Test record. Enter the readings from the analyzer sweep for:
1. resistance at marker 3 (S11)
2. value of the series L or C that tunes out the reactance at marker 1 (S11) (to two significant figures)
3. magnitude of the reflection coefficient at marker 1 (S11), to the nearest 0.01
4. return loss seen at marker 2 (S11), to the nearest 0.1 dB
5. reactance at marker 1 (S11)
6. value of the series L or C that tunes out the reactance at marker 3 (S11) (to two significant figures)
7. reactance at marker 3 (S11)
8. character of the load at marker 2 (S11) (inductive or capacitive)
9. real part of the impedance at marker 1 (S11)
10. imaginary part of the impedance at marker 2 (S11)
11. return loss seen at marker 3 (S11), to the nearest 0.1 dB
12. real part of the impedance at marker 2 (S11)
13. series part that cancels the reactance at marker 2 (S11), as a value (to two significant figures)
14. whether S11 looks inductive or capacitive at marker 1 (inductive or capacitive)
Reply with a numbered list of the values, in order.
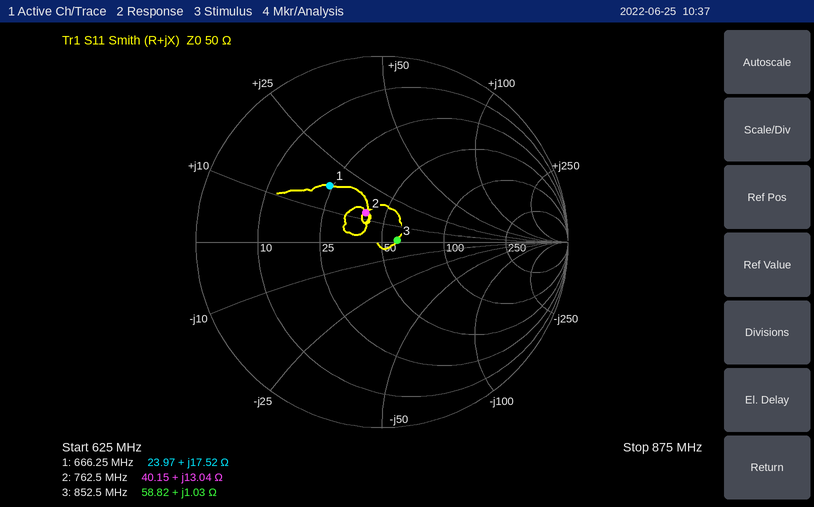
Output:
1. 58.82 Ω
2. 14 pF
3. 0.41
4. 14.9 dB
5. +17.52 Ω
6. 180 pF
7. +1.03 Ω
8. inductive
9. 23.97 Ω
10. +13.04 Ω
11. 21.8 dB
12. 40.15 Ω
13. 16 pF
14. inductive
